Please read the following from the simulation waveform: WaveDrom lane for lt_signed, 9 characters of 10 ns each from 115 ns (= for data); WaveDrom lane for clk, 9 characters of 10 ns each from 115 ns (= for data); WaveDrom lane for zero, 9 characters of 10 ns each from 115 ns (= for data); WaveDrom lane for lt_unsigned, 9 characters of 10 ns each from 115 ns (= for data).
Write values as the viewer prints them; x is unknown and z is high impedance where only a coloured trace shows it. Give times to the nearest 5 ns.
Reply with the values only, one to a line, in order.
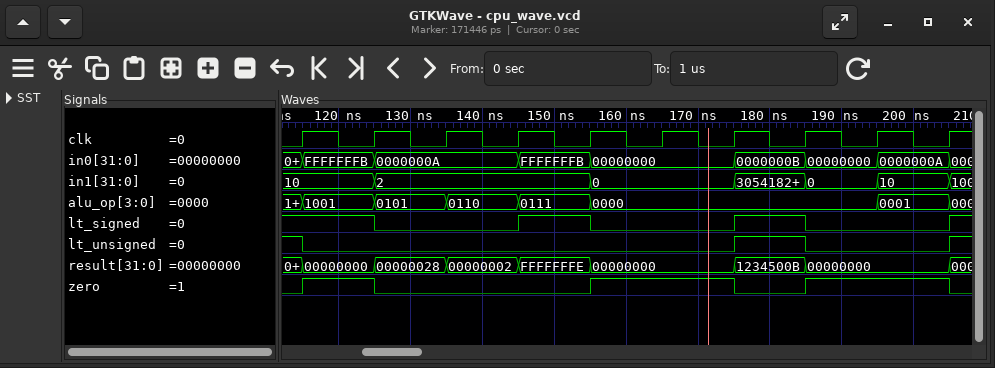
{name: 'lt_signed', wave: '10.10.10.'}
{name: 'clk', wave: 'p........'}
{name: 'zero', wave: '10..1.01.'}
{name: 'lt_unsigned', wave: '0.....10.'}
